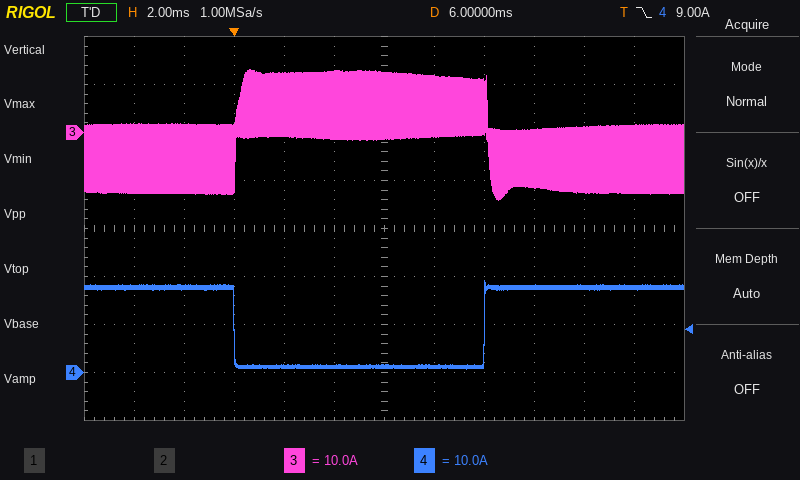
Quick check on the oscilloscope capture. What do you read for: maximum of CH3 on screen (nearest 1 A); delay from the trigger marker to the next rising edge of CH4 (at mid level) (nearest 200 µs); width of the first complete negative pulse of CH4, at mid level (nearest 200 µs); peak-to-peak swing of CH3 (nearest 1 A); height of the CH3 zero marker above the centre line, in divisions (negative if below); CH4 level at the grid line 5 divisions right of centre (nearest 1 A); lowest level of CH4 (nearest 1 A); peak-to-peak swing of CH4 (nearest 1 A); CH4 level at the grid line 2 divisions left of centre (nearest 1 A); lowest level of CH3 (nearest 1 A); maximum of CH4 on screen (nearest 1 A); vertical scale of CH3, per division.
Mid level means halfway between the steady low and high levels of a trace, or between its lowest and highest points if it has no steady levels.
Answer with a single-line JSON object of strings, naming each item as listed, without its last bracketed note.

{"maximum of CH3 on screen": "13 A", "delay from the trigger marker to the next rising edge of CH4 (at mid level)": "10.0 ms", "width of the first complete negative pulse of CH4, at mid level": "10.0 ms", "peak-to-peak swing of CH3": "27 A", "height of the CH3 zero marker above the centre line, in divisions": "+2.0 div", "CH4 level at the grid line 5 divisions right of centre": "18 A", "lowest level of CH4": "1 A", "peak-to-peak swing of CH4": "18 A", "CH4 level at the grid line 2 divisions left of centre": "1 A", "lowest level of CH3": "-14 A", "maximum of CH4 on screen": "19 A", "vertical scale of CH3, per division": "10 A"}
